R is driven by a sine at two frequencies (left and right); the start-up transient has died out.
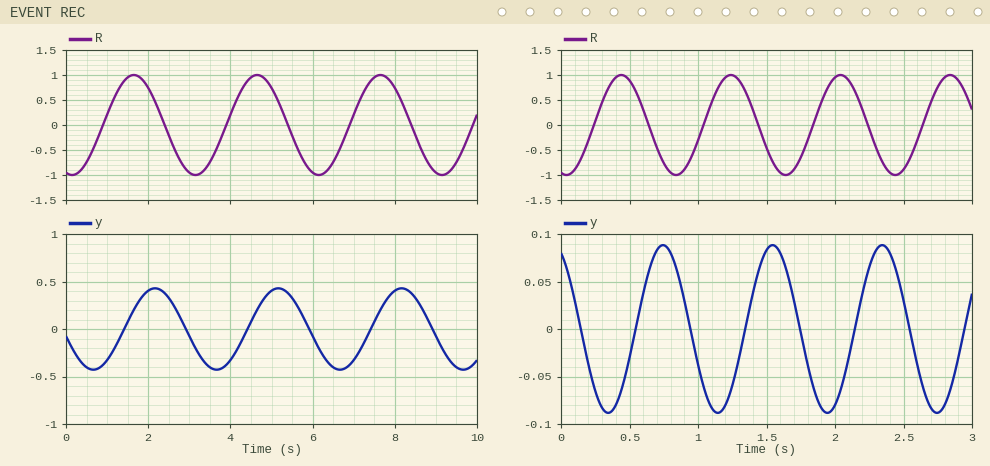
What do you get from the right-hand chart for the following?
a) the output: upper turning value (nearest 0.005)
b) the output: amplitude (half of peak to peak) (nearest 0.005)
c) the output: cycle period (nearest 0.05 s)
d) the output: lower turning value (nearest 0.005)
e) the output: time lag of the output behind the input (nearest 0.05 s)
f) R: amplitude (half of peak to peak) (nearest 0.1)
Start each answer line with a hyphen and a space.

- 0.090
- 0.090
- 0.80 s
- -0.090
- 0.30 s
- 1.0
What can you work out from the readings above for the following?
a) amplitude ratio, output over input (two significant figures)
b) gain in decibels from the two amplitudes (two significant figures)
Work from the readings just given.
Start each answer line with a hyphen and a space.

- 0.090
- -21 dB
